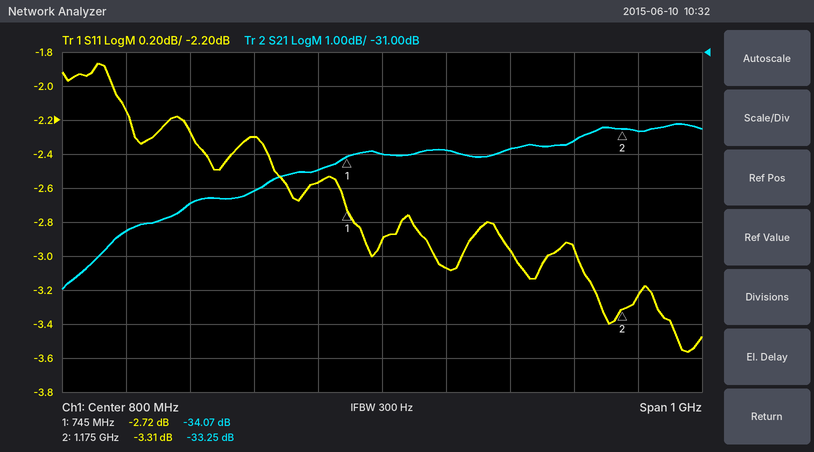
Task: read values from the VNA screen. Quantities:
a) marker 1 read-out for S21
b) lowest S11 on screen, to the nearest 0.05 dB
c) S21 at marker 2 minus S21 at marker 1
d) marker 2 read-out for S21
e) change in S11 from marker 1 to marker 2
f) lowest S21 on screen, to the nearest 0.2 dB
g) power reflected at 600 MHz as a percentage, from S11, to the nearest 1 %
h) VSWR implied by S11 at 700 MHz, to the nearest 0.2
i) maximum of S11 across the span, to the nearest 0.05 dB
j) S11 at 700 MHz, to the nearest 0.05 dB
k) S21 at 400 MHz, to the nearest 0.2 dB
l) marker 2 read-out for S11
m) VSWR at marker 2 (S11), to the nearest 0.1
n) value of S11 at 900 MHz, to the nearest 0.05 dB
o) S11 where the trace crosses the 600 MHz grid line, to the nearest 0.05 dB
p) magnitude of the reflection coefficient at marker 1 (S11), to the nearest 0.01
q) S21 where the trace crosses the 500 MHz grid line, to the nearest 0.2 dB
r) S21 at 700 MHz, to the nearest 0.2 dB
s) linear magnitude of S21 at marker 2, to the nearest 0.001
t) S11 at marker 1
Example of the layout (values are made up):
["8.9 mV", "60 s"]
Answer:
["-34.07 dB", "-3.55 dB", "0.82 dB", "-33.25 dB", "-0.59 dB", "-38.0 dB", "59 %", "6.8", "-1.85 dB", "-2.55 dB", "-36.2 dB", "-3.31 dB", "5.3", "-3.05 dB", "-2.30 dB", "0.73", "-35.4 dB", "-34.4 dB", "0.022", "-2.72 dB"]
